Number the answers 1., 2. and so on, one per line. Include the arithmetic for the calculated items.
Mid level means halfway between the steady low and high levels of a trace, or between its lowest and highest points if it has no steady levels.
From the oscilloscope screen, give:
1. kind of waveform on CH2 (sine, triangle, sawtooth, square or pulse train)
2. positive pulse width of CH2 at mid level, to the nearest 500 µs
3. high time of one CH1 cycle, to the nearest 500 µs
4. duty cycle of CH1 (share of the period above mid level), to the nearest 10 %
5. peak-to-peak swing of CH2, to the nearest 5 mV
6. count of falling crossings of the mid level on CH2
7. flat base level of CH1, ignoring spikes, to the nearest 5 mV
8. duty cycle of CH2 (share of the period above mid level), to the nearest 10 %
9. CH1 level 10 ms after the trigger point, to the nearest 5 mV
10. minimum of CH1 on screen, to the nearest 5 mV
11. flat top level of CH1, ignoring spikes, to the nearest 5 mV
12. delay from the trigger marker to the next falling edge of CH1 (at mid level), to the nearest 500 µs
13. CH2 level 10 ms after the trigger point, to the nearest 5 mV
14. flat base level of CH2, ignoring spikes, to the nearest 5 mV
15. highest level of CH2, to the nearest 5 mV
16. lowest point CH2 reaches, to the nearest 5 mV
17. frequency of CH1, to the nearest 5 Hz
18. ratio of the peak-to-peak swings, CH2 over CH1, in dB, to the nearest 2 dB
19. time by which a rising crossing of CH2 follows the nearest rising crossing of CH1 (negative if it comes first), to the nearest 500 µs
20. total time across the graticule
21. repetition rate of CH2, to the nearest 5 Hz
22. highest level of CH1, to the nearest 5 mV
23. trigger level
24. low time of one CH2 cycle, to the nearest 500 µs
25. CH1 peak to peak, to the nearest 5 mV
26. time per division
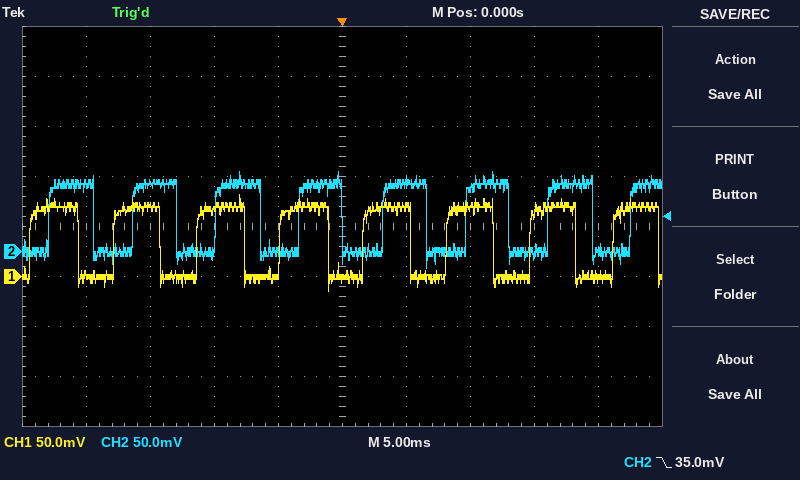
1. square
2. 3.5 ms
3. 3.5 ms
4. 60 %
5. 80 mV − (-15 mV) = 95 mV
6. 7
7. 0 mV
8. 50 %
9. 70 mV
10. -15 mV
11. 70 mV
12. 5.5 ms
13. 65 mV
14. 0 mV
15. 80 mV
16. -15 mV
17. 155 Hz
18. 20 log10(95 mV / 95 mV) ≈ 0 dB
19. +1.5 ms
20. 50 ms
21. 155 Hz
22. 80 mV
23. 35.0 mV
24. 3.0 ms
25. 80 mV − (-15 mV) = 95 mV
26. 5 ms
